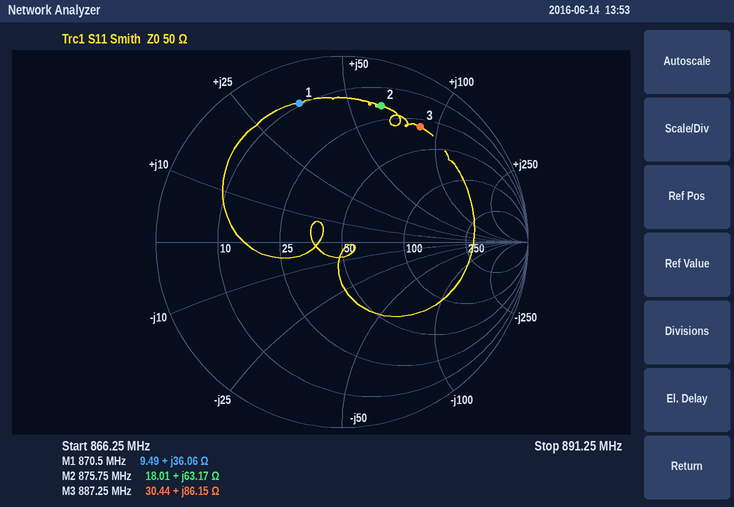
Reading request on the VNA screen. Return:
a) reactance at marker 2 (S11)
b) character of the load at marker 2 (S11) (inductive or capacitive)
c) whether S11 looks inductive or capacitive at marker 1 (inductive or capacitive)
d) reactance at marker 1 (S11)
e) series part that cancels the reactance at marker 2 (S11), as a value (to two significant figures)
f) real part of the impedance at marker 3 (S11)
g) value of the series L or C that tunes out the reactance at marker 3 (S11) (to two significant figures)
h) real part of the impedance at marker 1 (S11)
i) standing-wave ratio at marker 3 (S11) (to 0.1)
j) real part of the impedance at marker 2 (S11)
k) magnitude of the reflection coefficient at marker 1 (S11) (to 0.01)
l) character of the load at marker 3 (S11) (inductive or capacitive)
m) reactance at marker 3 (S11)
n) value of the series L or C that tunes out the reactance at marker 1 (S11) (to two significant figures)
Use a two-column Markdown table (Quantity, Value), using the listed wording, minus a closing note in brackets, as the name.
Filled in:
| Quantity | Value |
|---|---|
| reactance at marker 2 | +63.17 Ω |
| character of the load at marker 2 (S11) | inductive |
| whether S11 looks inductive or capacitive at marker 1 | inductive |
| reactance at marker 1 | +36.06 Ω |
| series part that cancels the reactance at marker 2 (S11), as a value | 2.9 pF |
| real part of the impedance at marker 3 | 30.44 Ω |
| value of the series L or C that tunes out the reactance at marker 3 (S11) | 2.1 pF |
| real part of the impedance at marker 1 | 9.49 Ω |
| standing-wave ratio at marker 3 (S11) | 7.0 |
| real part of the impedance at marker 2 | 18.01 Ω |
| magnitude of the reflection coefficient at marker 1 (S11) | 0.78 |
| character of the load at marker 3 (S11) | inductive |
| reactance at marker 3 | +86.15 Ω |
| value of the series L or C that tunes out the reactance at marker 1 (S11) | 5.1 pF |
